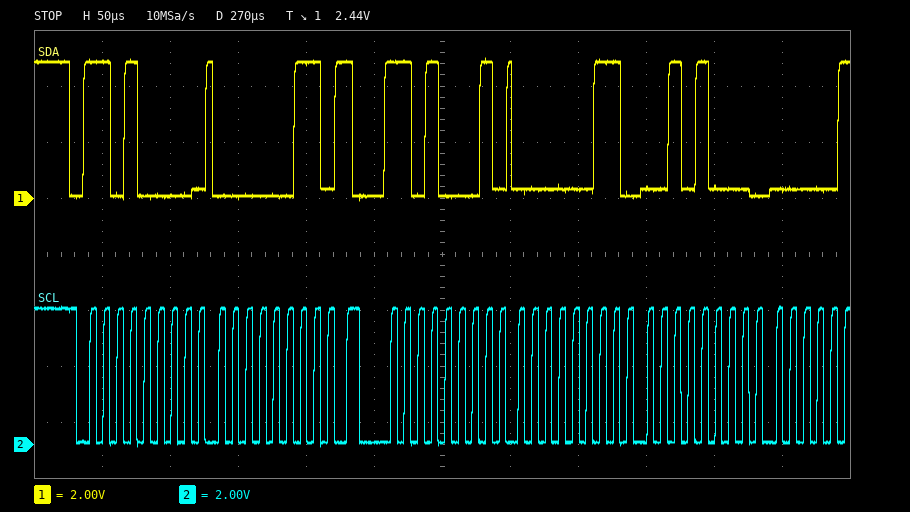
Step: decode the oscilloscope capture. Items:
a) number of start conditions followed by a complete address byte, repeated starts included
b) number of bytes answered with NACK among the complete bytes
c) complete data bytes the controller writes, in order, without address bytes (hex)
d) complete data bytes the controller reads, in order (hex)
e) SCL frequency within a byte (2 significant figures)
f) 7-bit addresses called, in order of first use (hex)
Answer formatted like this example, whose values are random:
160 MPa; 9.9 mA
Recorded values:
2; 0; 03; 03 28; 100 kHz; 0x68
